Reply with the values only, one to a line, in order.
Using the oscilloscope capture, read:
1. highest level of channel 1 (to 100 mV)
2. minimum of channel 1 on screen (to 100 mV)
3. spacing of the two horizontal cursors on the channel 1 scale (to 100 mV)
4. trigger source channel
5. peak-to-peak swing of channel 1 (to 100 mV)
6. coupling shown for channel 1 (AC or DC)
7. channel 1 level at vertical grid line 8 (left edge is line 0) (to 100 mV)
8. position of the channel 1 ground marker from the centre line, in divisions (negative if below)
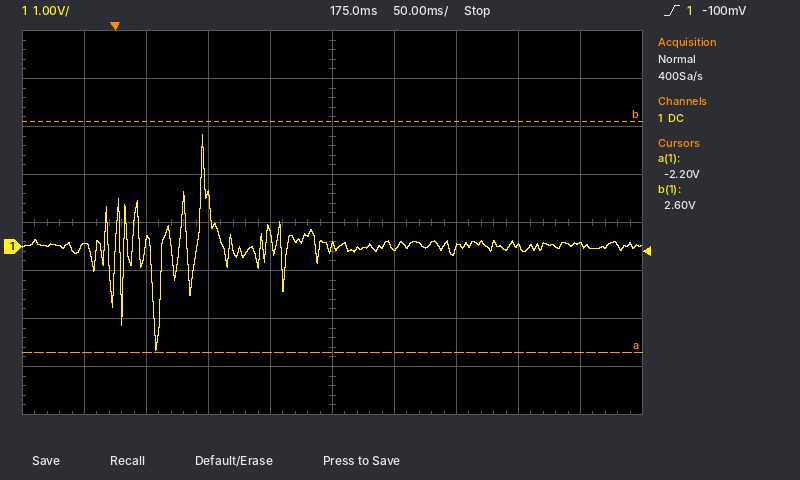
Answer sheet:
2.3 V
-2.2 V
4.8 V
channel 1
4.5 V
DC
0.0 V
-0.5 div
